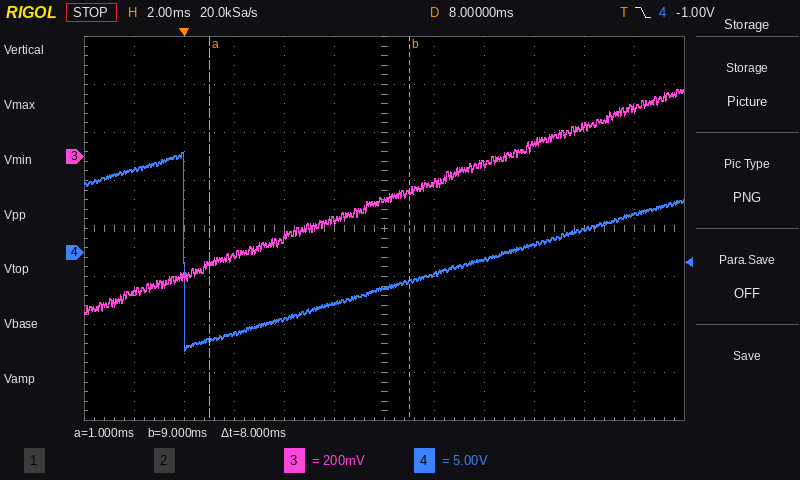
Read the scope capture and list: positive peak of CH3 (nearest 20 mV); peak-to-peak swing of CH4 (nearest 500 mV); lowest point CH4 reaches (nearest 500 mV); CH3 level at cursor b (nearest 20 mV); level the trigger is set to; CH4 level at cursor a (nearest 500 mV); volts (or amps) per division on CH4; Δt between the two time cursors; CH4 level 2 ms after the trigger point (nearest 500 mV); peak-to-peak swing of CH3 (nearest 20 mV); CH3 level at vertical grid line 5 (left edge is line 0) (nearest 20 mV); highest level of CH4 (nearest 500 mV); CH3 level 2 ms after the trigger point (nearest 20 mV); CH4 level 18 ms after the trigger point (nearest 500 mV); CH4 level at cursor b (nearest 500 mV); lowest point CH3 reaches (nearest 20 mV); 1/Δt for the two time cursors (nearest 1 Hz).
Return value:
280 mV
20.5 V
-10.0 V
-140 mV
-1.00 V
-9.0 V
5 V
8 ms
-8.5 V
940 mV
-260 mV
10.5 V
-400 mV
4.0 V
-3.0 V
-660 mV
125 Hz
